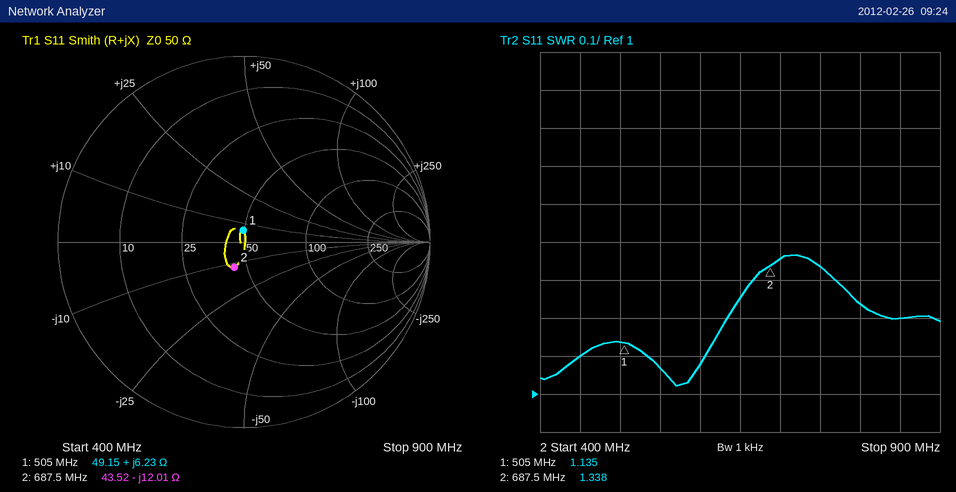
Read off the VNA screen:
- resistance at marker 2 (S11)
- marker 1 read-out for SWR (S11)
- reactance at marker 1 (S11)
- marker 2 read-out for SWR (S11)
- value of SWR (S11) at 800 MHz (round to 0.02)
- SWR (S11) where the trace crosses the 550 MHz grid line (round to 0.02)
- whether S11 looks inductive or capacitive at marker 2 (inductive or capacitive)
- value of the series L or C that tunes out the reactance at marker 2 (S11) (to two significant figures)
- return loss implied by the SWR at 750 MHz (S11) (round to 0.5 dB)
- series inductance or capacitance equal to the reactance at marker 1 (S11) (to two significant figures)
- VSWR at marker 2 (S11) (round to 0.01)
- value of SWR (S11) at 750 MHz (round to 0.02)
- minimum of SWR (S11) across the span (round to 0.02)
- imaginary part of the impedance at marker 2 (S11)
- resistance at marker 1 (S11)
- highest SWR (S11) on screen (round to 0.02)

43.52 Ω
1.135
+6.23 Ω
1.338
1.24
1.06
capacitive
2.8 nH
17.0 dB
2.0 nH
1.34
1.34
1.02
-12.01 Ω
49.15 Ω
1.36
